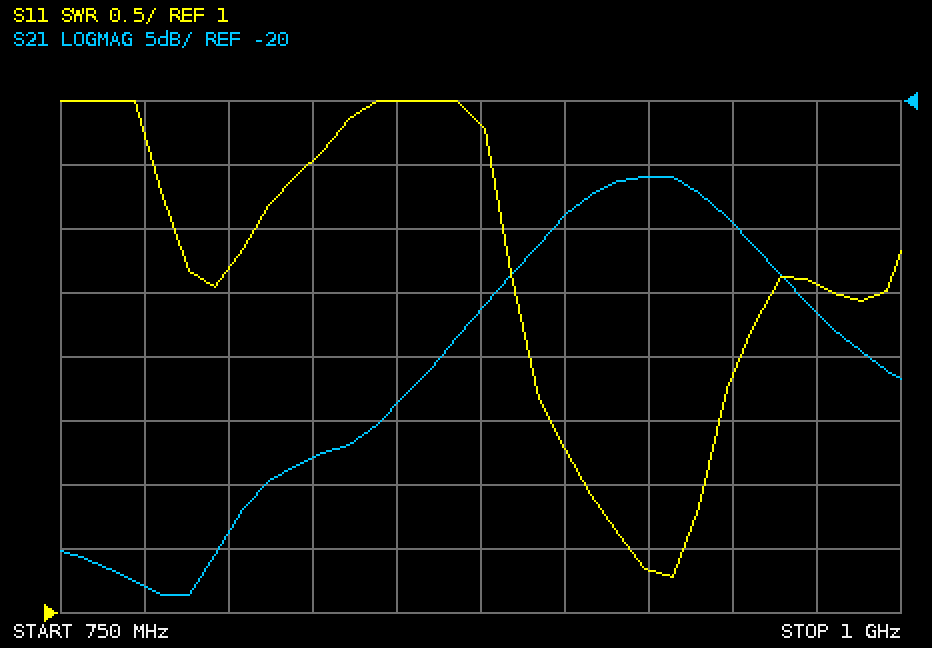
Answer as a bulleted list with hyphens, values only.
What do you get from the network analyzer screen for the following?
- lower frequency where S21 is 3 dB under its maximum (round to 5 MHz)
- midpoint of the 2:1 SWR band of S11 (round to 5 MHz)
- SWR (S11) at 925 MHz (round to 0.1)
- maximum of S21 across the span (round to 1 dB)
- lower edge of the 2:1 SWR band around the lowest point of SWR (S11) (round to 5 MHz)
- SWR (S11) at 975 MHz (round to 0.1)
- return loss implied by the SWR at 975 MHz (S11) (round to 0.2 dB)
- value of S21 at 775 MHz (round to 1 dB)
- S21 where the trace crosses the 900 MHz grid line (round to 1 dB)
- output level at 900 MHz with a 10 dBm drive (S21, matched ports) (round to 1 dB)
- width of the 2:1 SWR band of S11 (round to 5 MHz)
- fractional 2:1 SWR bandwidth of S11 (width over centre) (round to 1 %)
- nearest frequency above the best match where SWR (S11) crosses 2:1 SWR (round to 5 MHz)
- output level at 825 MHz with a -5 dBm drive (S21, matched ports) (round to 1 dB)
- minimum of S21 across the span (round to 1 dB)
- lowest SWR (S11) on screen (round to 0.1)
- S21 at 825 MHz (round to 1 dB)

- 900 MHz
- 925 MHz
- 1.3
- -26 dB
- 905 MHz
- 3.6
- 5.0 dB
- -58 dB
- -29 dB
- -19 dBm
- 35 MHz
- 4 %
- 940 MHz
- -53 dBm
- -59 dB
- 1.3
- -48 dB
